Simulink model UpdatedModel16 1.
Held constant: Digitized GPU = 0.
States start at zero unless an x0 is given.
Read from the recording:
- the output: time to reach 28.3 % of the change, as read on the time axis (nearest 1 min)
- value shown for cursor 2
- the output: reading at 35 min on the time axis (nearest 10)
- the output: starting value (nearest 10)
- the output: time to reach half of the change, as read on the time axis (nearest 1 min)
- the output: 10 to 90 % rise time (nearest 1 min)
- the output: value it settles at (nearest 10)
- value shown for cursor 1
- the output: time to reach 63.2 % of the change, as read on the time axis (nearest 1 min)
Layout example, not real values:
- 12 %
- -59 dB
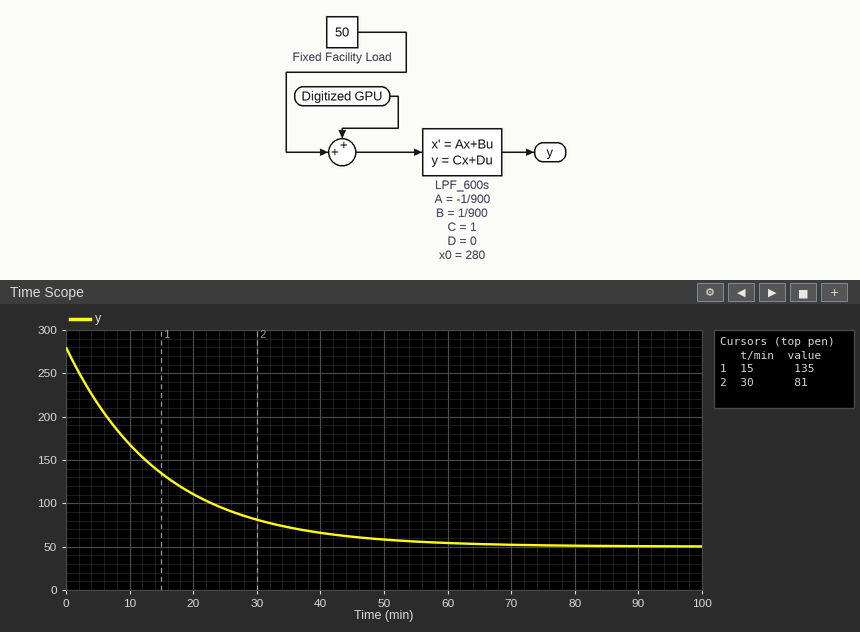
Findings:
- 5 min
- 81
- 70
- 280
- 10 min
- 33 min
- 50
- 135
- 15 min
